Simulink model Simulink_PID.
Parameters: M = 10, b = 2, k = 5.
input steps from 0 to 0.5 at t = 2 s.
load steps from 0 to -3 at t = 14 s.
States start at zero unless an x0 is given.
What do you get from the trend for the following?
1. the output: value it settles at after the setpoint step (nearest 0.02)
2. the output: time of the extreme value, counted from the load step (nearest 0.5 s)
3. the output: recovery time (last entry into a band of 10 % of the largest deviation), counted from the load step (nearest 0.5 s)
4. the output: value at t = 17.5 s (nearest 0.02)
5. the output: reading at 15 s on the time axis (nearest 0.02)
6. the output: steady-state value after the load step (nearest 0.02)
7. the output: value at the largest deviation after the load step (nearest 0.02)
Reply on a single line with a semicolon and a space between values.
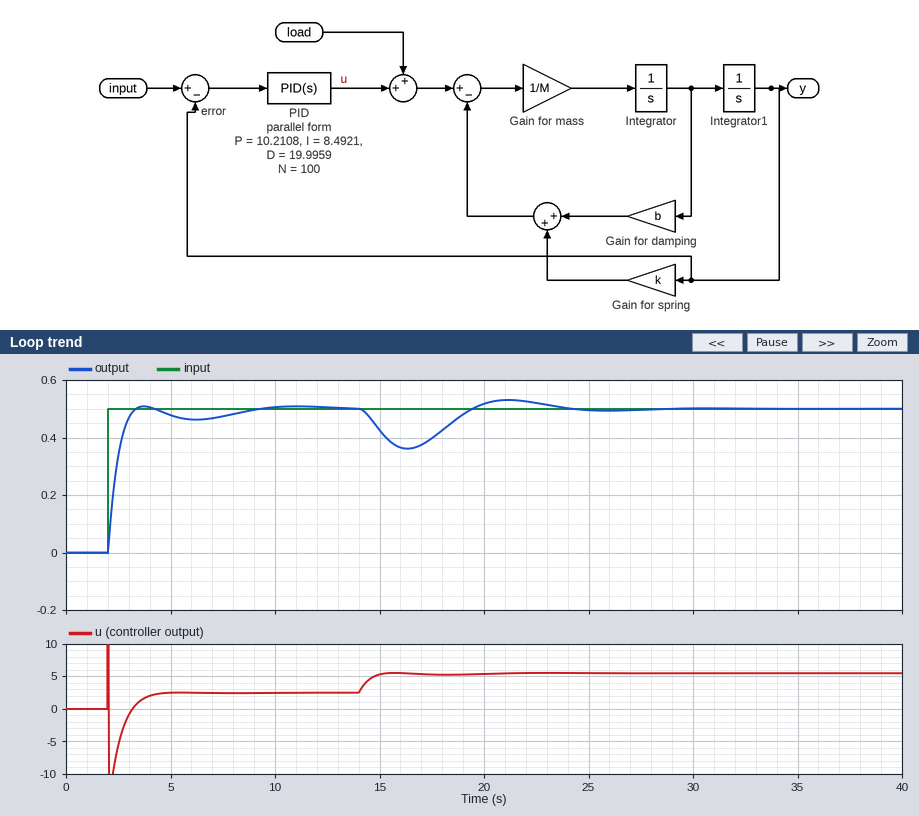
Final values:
0.50; 2.5 s; 9.0 s; 0.40; 0.42; 0.50; 0.36
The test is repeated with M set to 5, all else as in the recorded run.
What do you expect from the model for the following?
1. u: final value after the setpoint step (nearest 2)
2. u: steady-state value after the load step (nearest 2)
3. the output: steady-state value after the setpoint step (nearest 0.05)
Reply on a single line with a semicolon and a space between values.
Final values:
2; 6; 0.50
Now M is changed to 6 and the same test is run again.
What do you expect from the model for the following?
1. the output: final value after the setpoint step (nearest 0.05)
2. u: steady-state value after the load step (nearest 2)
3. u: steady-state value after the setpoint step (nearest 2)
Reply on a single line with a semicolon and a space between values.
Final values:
0.50; 6; 2
